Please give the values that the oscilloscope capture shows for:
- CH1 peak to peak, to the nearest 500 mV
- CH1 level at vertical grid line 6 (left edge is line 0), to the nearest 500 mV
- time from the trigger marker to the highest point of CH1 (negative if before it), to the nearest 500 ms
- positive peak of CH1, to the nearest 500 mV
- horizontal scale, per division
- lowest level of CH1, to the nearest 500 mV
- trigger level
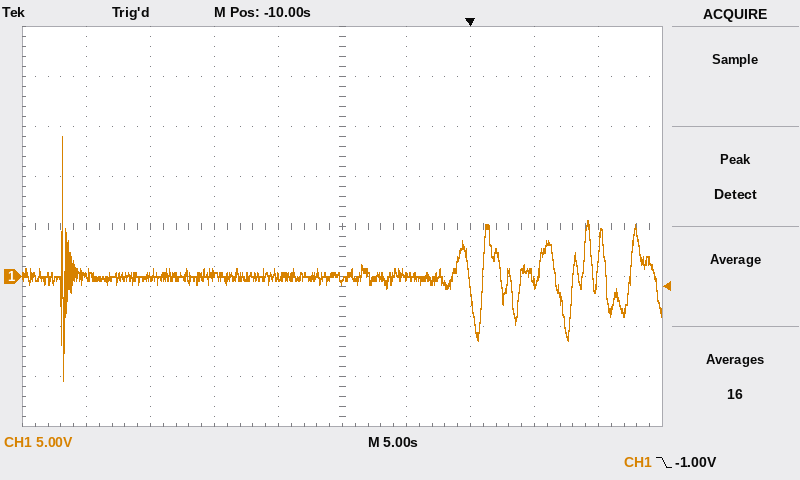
24.5 V
0.0 V
-32.0 s
14.0 V
5 s
-10.5 V
-1.00 V
